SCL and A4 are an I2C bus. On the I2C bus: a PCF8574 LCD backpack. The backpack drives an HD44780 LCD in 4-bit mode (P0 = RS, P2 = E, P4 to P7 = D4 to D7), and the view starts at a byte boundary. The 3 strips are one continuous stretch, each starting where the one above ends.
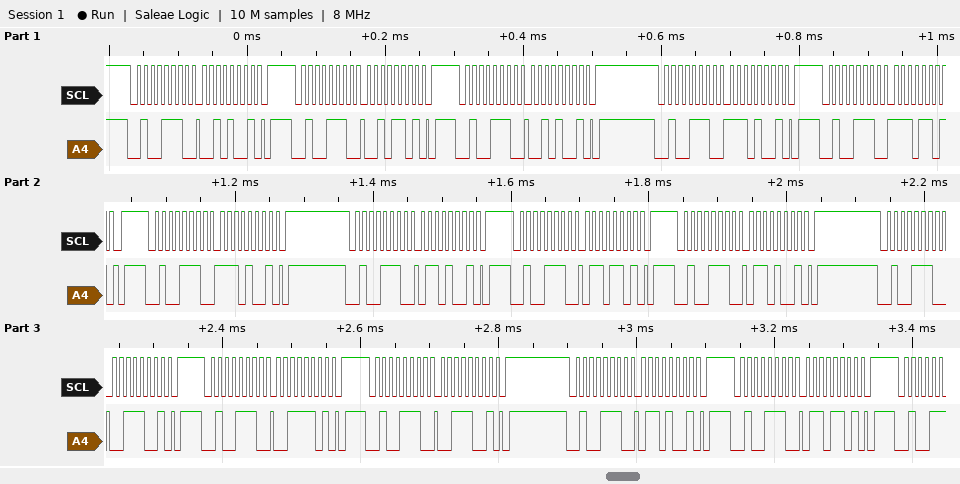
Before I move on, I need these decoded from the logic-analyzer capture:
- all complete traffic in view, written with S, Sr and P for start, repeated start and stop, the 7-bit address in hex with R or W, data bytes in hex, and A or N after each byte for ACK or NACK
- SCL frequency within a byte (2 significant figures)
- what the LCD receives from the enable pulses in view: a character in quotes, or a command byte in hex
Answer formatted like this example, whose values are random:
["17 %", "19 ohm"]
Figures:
["S 27W A 29 A P S 27W A 2D A P S 27W A 29 A P S 27W A E9 A P S 27W A ED A P S 27W A E9 A P S 27W A 69 A P S 27W A 6D A P S 27W A 69 A P S 27W A 39 A P S 27W A 3D A P S 27W A 39 A P S 27W A 69 A P S 27W A 6D A P", "100 kHz", "'.' 'c'"]
